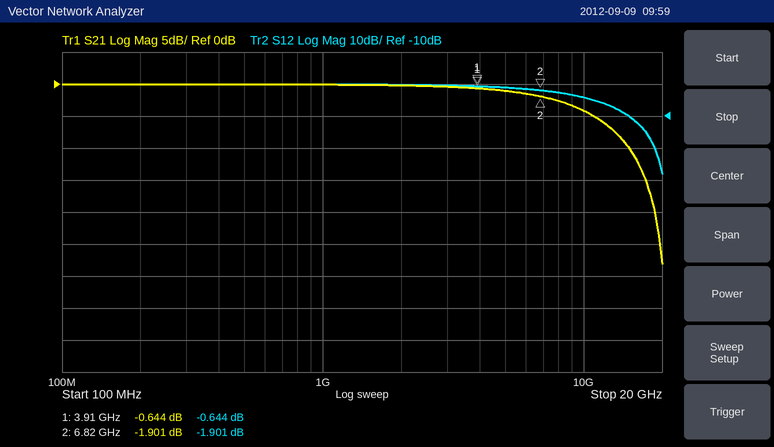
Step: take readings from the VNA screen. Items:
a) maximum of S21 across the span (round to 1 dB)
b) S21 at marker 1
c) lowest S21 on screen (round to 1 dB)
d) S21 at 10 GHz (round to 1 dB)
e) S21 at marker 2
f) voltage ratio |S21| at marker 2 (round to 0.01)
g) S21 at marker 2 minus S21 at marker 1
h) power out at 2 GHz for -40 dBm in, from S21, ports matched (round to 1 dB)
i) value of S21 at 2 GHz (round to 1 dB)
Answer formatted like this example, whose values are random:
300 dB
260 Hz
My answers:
0 dB
-0.644 dB
-28 dB
-4 dB
-1.901 dB
0.80
-1.257 dB
-40 dBm
0 dB
